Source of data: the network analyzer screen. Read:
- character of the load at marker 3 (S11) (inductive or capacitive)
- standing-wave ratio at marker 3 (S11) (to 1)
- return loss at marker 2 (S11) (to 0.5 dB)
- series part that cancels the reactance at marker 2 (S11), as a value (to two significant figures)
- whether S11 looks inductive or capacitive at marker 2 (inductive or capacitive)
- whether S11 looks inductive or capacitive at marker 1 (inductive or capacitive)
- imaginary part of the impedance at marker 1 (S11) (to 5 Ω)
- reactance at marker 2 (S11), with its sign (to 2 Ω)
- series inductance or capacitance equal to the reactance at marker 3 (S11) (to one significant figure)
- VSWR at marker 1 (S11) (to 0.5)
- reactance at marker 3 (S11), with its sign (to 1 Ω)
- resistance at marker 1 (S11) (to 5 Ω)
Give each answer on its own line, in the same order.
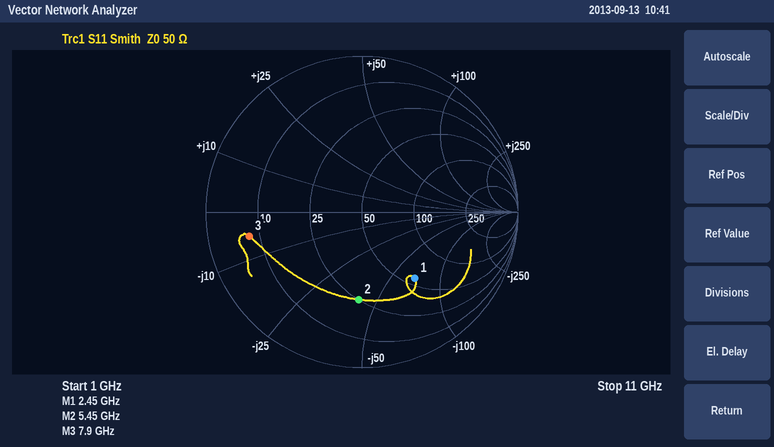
capacitive
7
5.0 dB
1.2 nH
capacitive
capacitive
-70 Ω
-42 Ω
4 pF
3.5
-5 Ω
55 Ω
